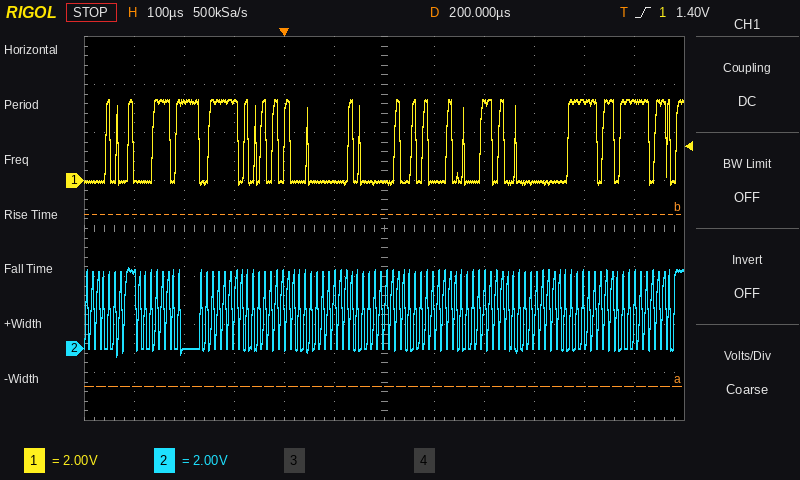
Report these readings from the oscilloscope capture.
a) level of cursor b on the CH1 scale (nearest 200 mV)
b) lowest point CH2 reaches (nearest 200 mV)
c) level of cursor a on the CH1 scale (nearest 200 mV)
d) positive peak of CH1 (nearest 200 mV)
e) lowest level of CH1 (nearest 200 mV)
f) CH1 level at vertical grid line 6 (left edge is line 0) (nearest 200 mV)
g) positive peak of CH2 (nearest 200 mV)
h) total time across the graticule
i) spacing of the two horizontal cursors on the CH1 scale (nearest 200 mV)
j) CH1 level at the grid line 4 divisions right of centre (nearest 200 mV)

-1.4 V
-400 mV
-8.6 V
3.4 V
-200 mV
0.0 V
3.4 V
1.2 ms
7.2 V
3.2 V
